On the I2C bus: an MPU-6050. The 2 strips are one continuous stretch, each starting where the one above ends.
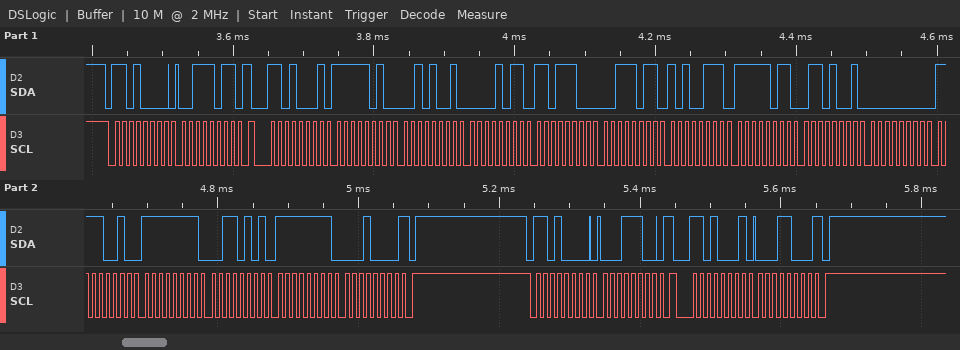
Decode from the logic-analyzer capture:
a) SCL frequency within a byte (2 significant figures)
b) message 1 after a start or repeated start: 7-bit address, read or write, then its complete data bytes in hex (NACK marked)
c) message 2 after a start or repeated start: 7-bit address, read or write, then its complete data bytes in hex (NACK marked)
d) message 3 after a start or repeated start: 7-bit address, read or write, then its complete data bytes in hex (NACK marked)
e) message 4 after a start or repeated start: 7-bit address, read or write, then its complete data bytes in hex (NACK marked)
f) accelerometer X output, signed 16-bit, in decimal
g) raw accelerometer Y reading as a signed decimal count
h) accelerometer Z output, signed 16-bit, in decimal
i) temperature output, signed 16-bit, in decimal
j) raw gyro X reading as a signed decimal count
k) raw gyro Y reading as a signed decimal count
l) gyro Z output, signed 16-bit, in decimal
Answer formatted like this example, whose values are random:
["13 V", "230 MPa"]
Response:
["100 kHz", "0x68 write: 3B", "0x68 read: FA 29 0B DC 3B A7 FB 69 00 F2 FF 35 FF 10 NACK", "0x68 write: 1C", "0x68 read: 18 NACK", "-1495", "3036", "15271", "-1175", "242", "-203", "-240"]
